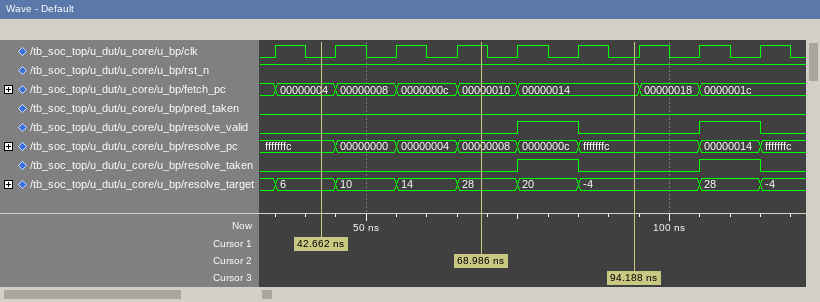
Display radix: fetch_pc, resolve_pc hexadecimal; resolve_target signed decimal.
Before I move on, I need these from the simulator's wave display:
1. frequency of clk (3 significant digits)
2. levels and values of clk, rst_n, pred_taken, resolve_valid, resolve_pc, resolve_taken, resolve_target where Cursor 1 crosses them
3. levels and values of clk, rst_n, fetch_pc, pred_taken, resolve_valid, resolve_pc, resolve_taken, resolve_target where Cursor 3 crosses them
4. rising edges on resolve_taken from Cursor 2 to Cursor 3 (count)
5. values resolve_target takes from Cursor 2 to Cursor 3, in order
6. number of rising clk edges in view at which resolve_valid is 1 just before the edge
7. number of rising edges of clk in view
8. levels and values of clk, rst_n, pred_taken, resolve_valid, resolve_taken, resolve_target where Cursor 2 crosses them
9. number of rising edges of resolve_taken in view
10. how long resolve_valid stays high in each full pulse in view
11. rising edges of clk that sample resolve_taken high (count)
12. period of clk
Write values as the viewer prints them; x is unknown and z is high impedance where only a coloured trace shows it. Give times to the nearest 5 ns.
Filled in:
100 MHz
clk=0, rst_n=1, pred_taken=0, resolve_valid=0, resolve_pc=fffffffc, resolve_taken=0, resolve_target=6
clk=0, rst_n=1, fetch_pc=00000014, pred_taken=0, resolve_valid=0, resolve_pc=fffffffc, resolve_taken=0, resolve_target=-4
1
28, 20, -4
2
9
clk=1, rst_n=1, pred_taken=0, resolve_valid=0, resolve_taken=0, resolve_target=28
2
10 ns, 10 ns
2
10 ns
